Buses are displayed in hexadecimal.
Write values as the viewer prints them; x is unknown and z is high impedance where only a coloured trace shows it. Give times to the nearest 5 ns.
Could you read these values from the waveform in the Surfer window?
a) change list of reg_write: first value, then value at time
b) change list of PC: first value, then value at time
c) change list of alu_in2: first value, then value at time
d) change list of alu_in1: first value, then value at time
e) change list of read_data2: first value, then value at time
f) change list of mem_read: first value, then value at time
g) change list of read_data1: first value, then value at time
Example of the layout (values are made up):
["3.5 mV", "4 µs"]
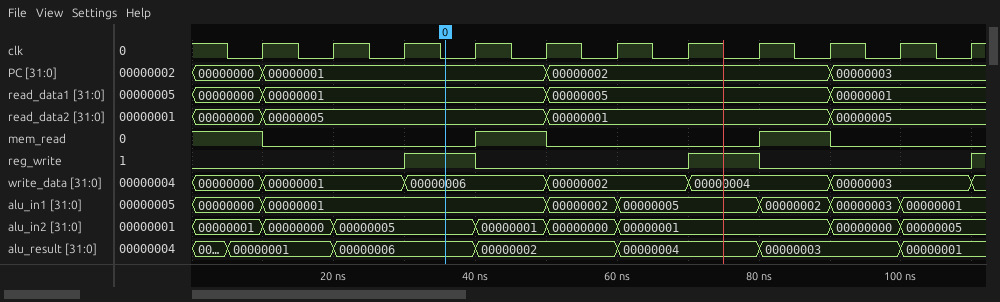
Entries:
["0, 1 at 30 ns, 0 at 40 ns, 1 at 70 ns, 0 at 80 ns, 1 at 110 ns", "00000000, 00000001 at 10 ns, 00000002 at 50 ns, 00000003 at 90 ns", "00000001, 00000000 at 10 ns, 00000005 at 20 ns, 00000001 at 40 ns, 00000000 at 50 ns, 00000001 at 60 ns, 00000000 at 90 ns, 00000005 at 100 ns", "00000000, 00000001 at 10 ns, 00000002 at 50 ns, 00000005 at 60 ns, 00000002 at 80 ns, 00000003 at 90 ns, 00000001 at 100 ns", "00000000, 00000005 at 10 ns, 00000001 at 50 ns, 00000005 at 90 ns", "1, 0 at 10 ns, 1 at 40 ns, 0 at 50 ns, 1 at 80 ns, 0 at 90 ns", "00000000, 00000001 at 10 ns, 00000005 at 50 ns, 00000001 at 90 ns"]
